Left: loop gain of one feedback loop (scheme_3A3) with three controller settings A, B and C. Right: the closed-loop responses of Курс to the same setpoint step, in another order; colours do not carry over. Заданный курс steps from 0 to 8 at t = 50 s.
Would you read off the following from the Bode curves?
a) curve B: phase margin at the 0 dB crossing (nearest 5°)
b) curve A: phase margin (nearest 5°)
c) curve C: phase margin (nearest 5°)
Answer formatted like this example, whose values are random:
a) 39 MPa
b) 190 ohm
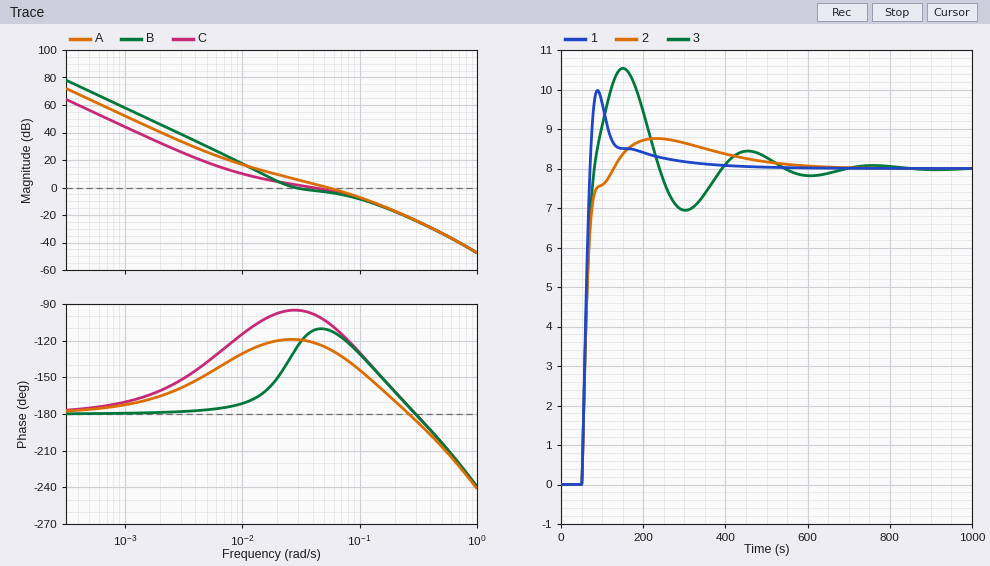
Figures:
a) 50°
b) 55°
c) 80°
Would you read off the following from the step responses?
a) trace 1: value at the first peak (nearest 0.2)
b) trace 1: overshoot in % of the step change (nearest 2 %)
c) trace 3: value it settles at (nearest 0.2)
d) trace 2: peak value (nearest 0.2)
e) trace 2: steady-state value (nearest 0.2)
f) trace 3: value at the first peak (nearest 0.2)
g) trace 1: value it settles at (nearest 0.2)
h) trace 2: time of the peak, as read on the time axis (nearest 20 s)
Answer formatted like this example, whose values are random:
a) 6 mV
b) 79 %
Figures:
a) 10.0
b) 24 %
c) 8.0
d) 8.8
e) 8.0
f) 10.6
g) 8.0
h) 240 s
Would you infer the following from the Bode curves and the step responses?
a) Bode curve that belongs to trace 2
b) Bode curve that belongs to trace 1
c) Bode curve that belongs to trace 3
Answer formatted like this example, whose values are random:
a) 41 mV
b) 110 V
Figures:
a) C
b) A
c) B
